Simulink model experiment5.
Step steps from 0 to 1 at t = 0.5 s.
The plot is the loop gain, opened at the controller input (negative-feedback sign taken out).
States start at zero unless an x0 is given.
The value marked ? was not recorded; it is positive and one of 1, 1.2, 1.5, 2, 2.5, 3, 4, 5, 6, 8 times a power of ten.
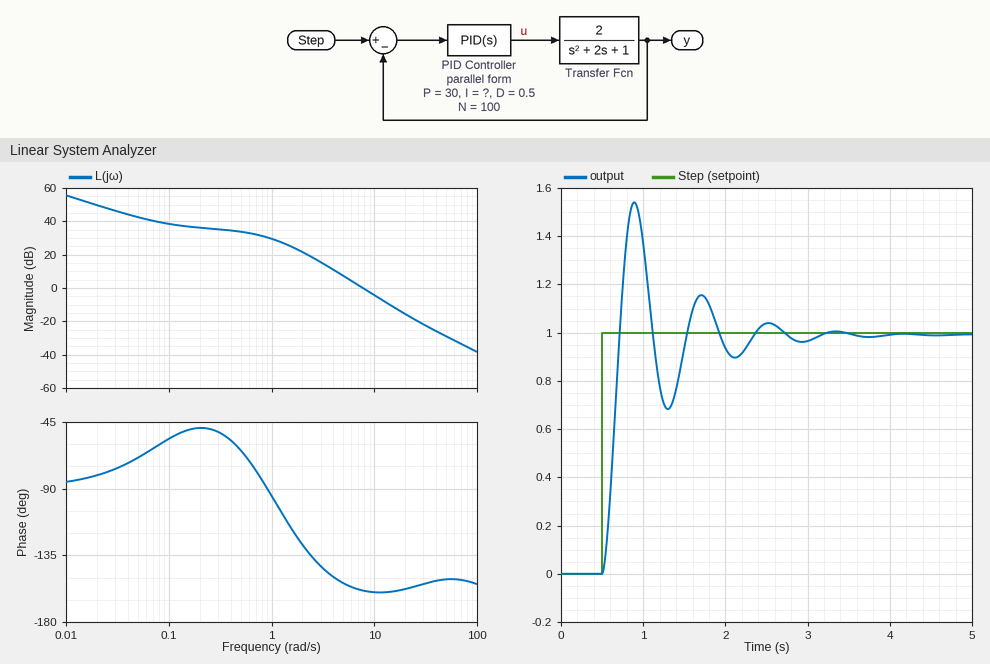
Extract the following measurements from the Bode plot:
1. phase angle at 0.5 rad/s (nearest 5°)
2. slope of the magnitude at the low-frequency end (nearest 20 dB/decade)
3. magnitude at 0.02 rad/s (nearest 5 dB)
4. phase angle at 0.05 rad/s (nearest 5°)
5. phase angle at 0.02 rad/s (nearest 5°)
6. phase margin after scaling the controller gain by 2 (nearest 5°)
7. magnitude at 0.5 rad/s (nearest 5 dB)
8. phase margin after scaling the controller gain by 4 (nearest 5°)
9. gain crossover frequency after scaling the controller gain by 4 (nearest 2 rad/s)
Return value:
-65°
-20 dB/decade
50 dB
-70°
-80°
20°
35 dB
20°
16 rad/s
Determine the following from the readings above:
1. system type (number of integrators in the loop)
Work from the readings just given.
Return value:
1
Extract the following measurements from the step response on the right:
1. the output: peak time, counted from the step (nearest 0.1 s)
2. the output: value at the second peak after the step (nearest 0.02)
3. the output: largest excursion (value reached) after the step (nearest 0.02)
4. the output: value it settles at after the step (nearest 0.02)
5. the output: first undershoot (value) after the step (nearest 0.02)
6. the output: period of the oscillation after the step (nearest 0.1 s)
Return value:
0.4 s
1.16
1.54
1.00
0.68
0.8 s
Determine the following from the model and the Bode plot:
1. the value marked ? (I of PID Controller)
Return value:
3
